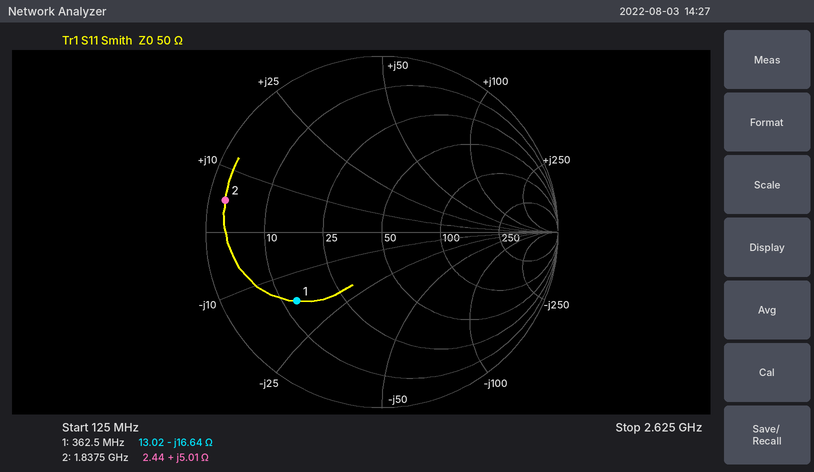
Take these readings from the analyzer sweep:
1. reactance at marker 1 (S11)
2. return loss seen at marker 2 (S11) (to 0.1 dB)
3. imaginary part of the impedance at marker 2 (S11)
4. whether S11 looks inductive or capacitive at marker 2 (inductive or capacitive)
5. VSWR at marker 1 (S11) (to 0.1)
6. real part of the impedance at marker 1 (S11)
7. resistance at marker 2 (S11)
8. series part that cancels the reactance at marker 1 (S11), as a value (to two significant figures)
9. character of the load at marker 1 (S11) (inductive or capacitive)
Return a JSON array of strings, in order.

["-16.64 Ω", "0.8 dB", "+5.01 Ω", "inductive", "4.3", "13.02 Ω", "2.44 Ω", "7.3 nH", "capacitive"]
